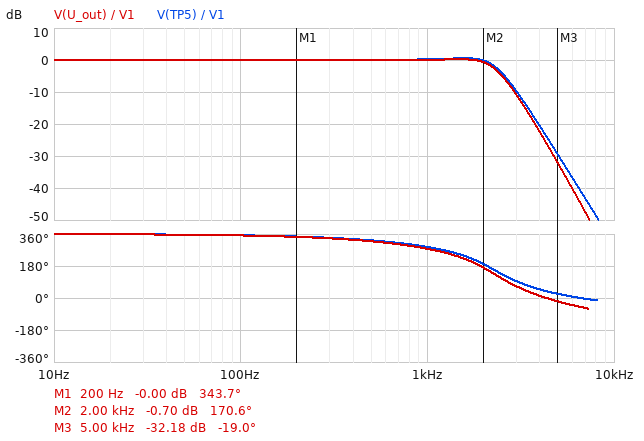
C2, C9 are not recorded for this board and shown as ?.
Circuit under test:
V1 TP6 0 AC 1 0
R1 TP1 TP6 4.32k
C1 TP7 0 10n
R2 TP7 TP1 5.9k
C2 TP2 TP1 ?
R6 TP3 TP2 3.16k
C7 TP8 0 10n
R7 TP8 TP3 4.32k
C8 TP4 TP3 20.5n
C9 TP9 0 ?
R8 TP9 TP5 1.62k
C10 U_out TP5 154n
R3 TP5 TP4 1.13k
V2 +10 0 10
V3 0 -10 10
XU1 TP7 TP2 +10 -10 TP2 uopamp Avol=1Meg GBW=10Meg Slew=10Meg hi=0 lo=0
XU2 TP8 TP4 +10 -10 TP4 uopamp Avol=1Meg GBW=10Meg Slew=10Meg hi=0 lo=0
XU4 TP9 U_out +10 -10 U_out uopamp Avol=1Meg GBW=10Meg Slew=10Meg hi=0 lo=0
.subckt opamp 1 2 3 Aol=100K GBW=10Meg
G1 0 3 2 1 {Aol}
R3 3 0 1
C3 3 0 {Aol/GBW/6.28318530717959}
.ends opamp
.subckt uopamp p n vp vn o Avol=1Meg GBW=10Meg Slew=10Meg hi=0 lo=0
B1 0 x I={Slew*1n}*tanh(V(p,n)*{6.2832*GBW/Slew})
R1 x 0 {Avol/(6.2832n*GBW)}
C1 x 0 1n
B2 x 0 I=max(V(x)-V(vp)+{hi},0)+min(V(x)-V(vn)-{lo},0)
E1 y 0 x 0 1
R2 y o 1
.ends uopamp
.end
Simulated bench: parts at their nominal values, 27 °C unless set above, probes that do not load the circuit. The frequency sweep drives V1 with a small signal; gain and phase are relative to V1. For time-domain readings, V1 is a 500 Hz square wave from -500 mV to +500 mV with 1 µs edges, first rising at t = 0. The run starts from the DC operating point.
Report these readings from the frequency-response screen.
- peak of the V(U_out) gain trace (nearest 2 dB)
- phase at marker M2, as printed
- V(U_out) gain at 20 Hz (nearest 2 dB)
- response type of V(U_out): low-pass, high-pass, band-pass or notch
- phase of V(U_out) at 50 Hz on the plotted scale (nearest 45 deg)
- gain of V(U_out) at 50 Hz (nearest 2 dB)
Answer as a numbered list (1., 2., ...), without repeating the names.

1. 0 dB
2. 170.6 deg
3. 0 dB
4. low-pass
5. 360 deg
6. 0 dB
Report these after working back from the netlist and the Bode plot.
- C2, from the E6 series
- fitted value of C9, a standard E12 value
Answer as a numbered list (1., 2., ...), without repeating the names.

1. 4.7 nF
2. 18 nF
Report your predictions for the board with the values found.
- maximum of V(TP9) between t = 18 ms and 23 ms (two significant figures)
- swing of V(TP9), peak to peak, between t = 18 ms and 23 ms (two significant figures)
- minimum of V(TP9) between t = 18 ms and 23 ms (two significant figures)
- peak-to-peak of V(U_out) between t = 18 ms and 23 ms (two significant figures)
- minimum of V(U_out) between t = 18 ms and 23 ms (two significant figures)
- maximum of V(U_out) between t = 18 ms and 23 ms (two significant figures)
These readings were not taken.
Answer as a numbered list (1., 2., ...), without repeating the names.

1. 630 mV
2. 1.3 V
3. -630 mV
4. 1.3 V
5. -630 mV
6. 630 mV
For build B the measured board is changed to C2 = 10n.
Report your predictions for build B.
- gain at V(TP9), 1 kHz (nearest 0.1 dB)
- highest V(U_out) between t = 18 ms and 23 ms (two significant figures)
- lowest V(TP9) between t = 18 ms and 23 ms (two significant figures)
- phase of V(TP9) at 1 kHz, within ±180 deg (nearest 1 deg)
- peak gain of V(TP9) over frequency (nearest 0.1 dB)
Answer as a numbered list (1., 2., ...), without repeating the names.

1. 0.4 dB
2. 670 mV
3. -670 mV
4. -85 deg
5. 0.8 dB
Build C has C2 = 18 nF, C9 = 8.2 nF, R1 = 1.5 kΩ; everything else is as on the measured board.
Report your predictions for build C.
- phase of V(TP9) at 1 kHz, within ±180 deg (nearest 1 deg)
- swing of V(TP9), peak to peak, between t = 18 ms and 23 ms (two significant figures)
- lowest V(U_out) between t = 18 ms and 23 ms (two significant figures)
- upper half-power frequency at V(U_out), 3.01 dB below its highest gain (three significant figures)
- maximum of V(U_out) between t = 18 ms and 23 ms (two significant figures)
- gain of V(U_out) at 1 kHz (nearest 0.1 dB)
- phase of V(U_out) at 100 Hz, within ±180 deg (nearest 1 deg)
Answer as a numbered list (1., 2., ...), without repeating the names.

1. -63 deg
2. 1.4 V
3. -700 mV
4. 3.39 kHz
5. 700 mV
6. 0.3 dB
7. -6 deg
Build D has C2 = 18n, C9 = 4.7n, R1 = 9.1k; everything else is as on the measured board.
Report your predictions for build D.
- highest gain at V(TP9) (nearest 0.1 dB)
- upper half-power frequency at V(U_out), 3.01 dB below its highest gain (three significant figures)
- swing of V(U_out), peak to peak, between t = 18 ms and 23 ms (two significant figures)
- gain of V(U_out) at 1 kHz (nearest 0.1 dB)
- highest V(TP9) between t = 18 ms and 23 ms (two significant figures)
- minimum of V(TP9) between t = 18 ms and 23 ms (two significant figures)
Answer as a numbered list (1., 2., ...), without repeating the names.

1. 0 dB
2. 1.66 kHz
3. 1.1 V
4. -0.7 dB
5. 540 mV
6. -540 mV
